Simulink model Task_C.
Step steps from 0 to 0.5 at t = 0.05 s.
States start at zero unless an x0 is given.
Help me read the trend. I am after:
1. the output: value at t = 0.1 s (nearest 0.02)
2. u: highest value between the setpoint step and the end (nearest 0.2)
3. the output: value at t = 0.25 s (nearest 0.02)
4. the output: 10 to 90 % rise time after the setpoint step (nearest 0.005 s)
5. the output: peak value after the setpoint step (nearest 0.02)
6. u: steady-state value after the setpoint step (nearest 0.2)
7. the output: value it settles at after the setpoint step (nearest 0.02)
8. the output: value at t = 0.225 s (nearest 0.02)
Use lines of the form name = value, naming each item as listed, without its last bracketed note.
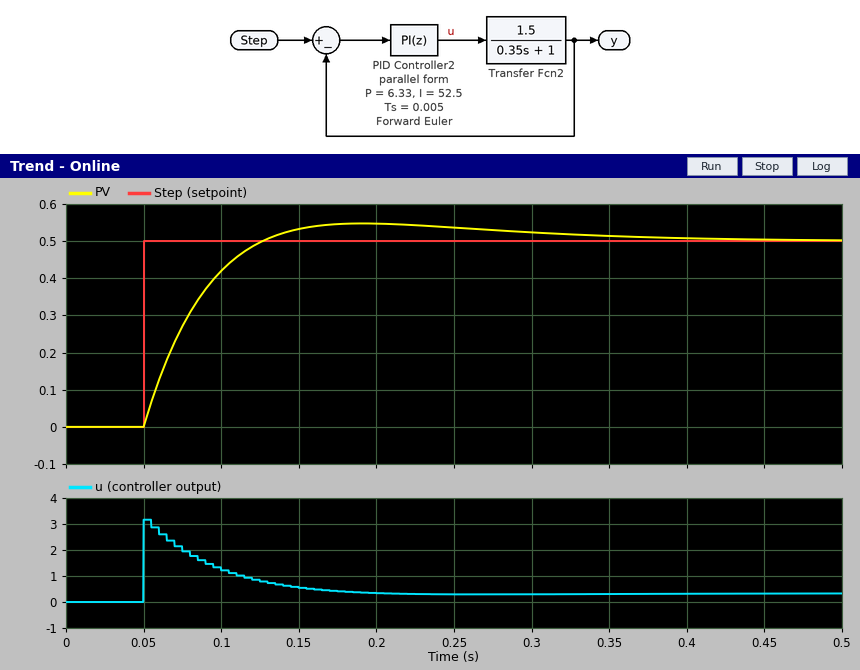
the output: value at t = 0.1 s = 0.42
u: highest value between the setpoint step and the end = 3.2
the output: value at t = 0.25 s = 0.54
the output: 10 to 90 % rise time after the setpoint step = 0.055 s
the output: peak value after the setpoint step = 0.54
u: steady-state value after the setpoint step = 0.4
the output: value it settles at after the setpoint step = 0.50
the output: value at t = 0.225 s = 0.54
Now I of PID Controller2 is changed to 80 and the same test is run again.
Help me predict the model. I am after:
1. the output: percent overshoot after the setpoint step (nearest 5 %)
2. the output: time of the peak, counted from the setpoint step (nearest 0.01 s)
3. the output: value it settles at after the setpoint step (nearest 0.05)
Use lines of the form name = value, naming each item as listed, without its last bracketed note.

the output: percent overshoot after the setpoint step = 15 %
the output: time of the peak, counted from the setpoint step = 0.12 s
the output: value it settles at after the setpoint step = 0.50
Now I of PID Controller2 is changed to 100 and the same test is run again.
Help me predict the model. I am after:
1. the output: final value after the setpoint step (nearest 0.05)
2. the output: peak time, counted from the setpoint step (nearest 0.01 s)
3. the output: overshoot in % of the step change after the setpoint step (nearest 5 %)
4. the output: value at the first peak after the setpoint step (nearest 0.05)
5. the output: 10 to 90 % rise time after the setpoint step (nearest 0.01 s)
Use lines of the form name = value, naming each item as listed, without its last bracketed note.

the output: final value after the setpoint step = 0.50
the output: peak time, counted from the setpoint step = 0.11 s
the output: overshoot in % of the step change after the setpoint step = 20 %
the output: value at the first peak after the setpoint step = 0.60
the output: 10 to 90 % rise time after the setpoint step = 0.04 s
